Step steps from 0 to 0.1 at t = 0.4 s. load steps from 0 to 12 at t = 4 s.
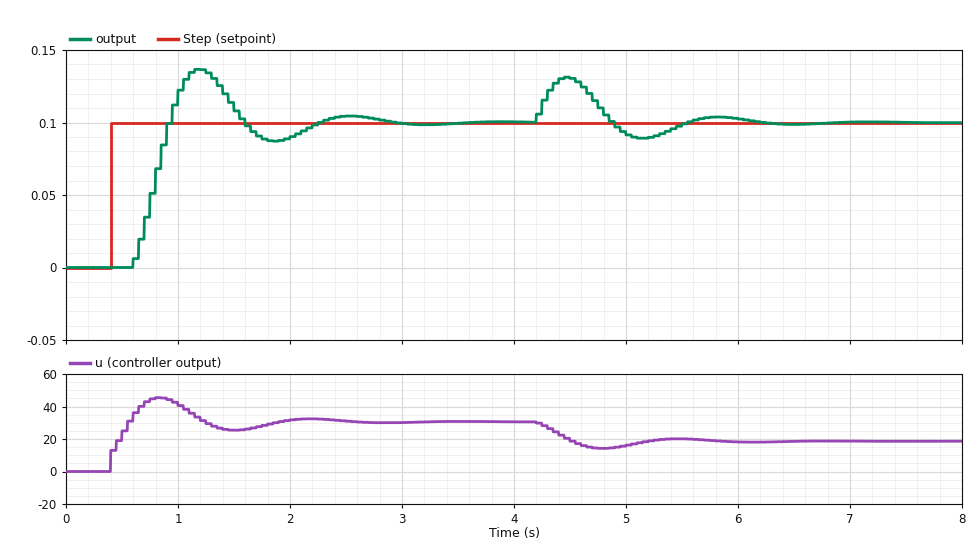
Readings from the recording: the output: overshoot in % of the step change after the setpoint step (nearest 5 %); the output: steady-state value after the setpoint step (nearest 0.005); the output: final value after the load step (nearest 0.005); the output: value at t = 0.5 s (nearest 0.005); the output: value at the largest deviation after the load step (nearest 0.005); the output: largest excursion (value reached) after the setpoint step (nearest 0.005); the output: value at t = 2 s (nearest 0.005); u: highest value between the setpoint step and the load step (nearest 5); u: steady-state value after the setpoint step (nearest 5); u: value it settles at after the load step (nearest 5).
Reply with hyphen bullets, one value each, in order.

- 35 %
- 0.100
- 0.100
- 0.000
- 0.130
- 0.135
- 0.090
- 45
- 30
- 20
